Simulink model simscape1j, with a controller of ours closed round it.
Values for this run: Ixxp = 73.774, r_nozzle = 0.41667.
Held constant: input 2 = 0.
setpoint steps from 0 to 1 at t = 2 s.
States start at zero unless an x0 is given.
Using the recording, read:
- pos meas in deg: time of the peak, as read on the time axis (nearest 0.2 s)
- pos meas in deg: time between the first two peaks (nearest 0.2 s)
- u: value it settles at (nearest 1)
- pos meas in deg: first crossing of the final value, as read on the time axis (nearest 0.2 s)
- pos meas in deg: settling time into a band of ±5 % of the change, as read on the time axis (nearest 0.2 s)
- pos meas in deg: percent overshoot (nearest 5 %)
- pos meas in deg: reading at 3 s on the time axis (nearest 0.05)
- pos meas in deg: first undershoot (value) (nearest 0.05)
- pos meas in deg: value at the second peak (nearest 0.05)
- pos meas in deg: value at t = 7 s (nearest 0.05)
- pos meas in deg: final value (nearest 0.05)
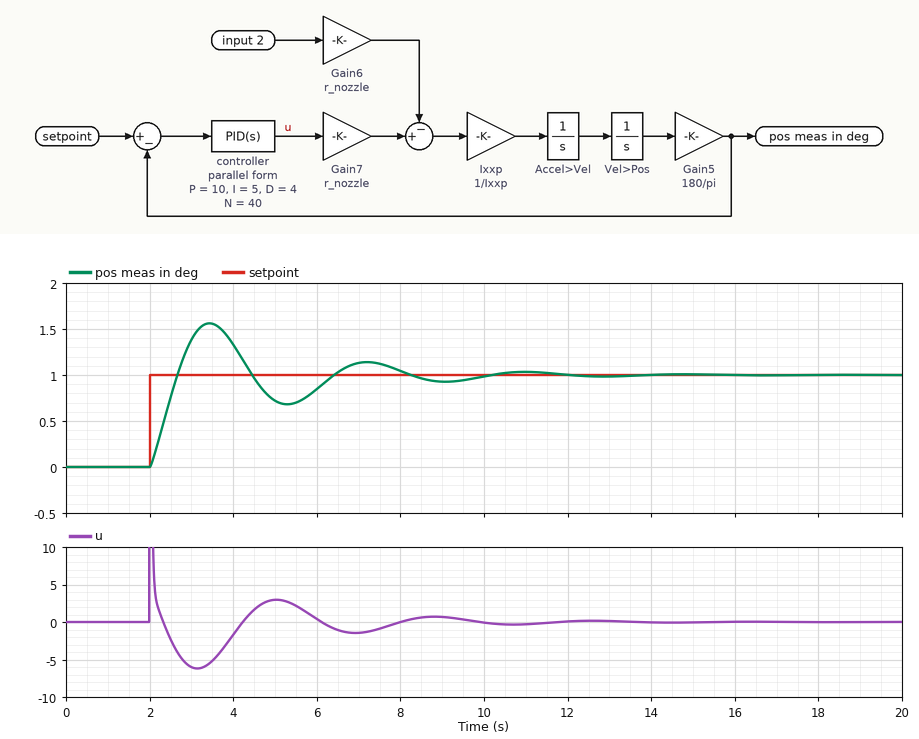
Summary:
3.4 s
3.8 s
0
2.6 s
9.6 s
55 %
1.40
0.70
1.15
1.15
1.00
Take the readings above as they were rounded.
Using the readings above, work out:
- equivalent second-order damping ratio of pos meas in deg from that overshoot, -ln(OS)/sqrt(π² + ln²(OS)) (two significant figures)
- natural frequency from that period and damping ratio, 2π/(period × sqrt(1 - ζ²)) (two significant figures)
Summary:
0.19
1.7 rad/s
